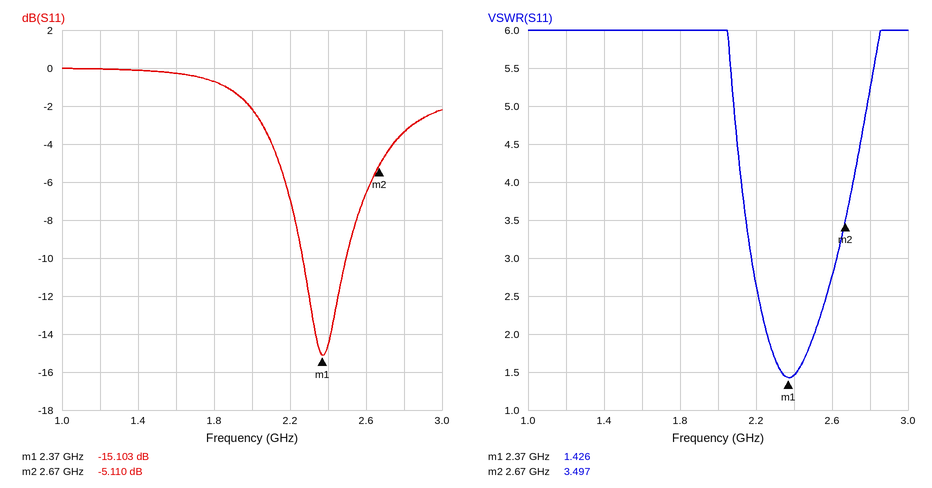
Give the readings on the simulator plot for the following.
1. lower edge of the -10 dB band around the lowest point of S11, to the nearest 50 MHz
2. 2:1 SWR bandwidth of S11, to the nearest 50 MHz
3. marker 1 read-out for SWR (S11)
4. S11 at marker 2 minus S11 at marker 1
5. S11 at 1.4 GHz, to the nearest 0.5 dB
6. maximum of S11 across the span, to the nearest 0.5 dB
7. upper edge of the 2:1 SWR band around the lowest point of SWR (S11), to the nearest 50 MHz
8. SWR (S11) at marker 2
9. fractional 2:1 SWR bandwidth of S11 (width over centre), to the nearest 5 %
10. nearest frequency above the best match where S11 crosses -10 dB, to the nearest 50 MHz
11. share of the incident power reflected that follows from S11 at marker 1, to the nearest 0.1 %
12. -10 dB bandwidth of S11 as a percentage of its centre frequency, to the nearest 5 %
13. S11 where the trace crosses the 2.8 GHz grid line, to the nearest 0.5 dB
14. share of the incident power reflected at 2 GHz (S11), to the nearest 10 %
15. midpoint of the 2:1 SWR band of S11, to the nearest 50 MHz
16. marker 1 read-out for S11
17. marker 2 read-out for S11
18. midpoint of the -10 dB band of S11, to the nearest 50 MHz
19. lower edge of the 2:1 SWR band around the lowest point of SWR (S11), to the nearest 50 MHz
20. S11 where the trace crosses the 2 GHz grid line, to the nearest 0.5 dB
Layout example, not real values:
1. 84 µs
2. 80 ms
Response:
1. 2.25 GHz
2. 250 MHz
3. 1.426
4. 9.993 dB
5. 0.0 dB
6. 0.0 dB
7. 2.50 GHz
8. 3.497
9. 10 %
10. 2.50 GHz
11. 3.1 %
12. 10 %
13. -3.5 dB
14. 60 %
15. 2.40 GHz
16. -15.103 dB
17. -5.110 dB
18. 2.40 GHz
19. 2.25 GHz
20. -2.0 dB
